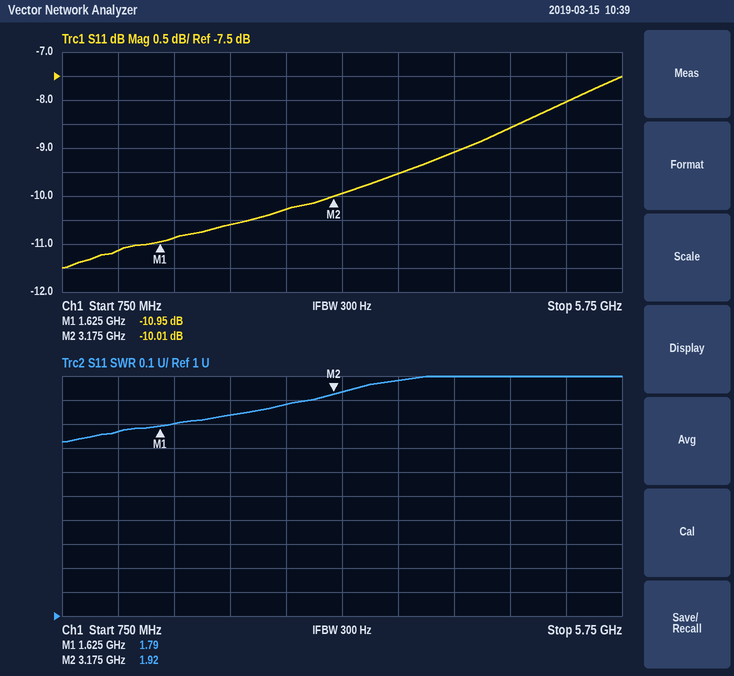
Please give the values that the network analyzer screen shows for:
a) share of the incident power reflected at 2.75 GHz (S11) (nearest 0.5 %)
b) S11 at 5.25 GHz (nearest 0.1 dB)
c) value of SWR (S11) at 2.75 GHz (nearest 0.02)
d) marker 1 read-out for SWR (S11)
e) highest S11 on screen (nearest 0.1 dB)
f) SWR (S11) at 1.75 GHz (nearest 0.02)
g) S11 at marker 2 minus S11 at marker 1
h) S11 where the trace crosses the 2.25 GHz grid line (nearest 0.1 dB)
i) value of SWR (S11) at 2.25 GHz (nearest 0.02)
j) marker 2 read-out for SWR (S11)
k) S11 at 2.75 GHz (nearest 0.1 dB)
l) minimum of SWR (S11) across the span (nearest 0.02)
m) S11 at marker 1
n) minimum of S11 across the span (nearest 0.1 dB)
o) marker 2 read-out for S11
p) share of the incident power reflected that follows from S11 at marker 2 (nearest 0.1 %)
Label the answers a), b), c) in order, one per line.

a) 9.5 %
b) -8.0 dB
c) 1.88
d) 1.79
e) -7.5 dB
f) 1.80
g) 0.94 dB
h) -10.6 dB
i) 1.84
j) 1.92
k) -10.3 dB
l) 1.72
m) -10.95 dB
n) -11.5 dB
o) -10.01 dB
p) 10.0 %
